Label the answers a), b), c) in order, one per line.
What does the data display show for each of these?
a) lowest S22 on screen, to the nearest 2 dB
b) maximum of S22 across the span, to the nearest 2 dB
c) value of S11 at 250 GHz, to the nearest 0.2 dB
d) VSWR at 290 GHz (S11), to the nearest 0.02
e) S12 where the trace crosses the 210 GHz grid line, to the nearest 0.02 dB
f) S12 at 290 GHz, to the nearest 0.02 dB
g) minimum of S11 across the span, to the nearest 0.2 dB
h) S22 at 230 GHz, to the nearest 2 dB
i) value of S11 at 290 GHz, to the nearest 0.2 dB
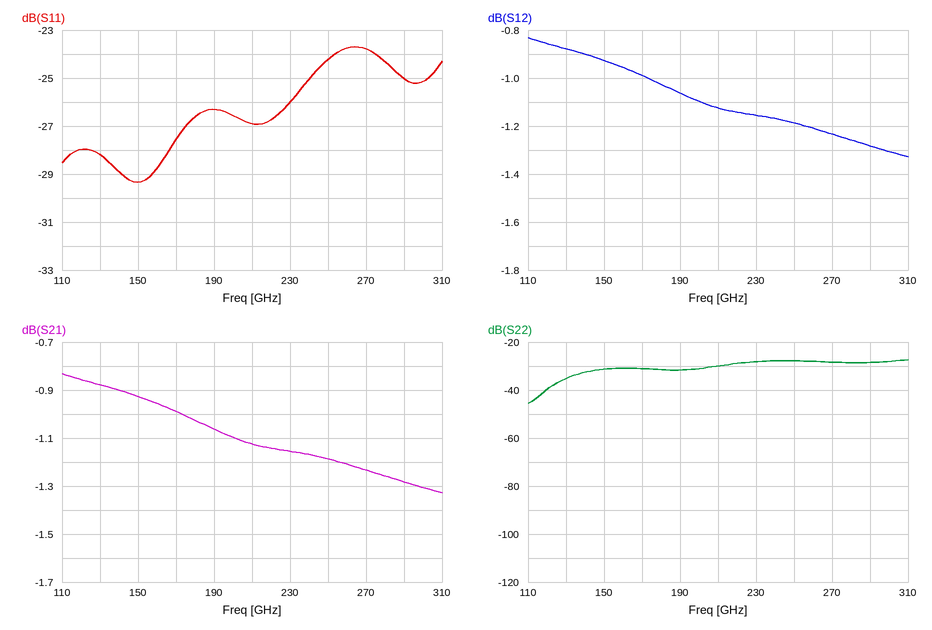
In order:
a) -46 dB
b) -28 dB
c) -24.2 dB
d) 1.12
e) -1.12 dB
f) -1.28 dB
g) -29.4 dB
h) -28 dB
i) -25.0 dB
